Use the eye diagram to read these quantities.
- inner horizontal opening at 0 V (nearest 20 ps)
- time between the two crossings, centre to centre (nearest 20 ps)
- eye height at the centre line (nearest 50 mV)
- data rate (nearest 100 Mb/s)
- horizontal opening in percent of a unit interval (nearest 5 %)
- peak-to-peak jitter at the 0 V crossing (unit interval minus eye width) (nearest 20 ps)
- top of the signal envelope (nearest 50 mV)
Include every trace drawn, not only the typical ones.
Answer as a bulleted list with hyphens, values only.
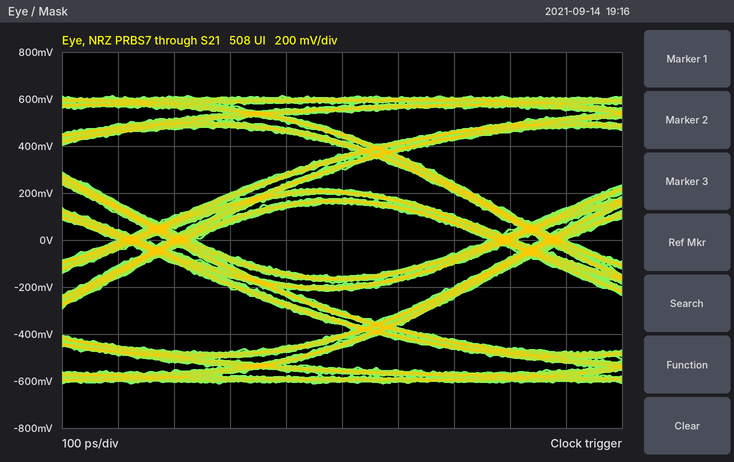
- 520 ps
- 660 ps
- 300 mV
- 1.5 Gb/s
- 80 %
- 140 ps
- 600 mV
